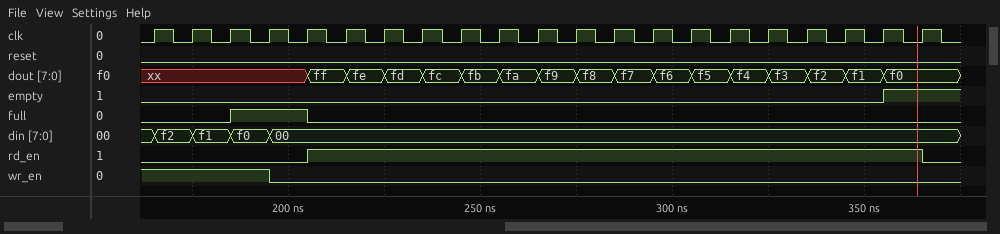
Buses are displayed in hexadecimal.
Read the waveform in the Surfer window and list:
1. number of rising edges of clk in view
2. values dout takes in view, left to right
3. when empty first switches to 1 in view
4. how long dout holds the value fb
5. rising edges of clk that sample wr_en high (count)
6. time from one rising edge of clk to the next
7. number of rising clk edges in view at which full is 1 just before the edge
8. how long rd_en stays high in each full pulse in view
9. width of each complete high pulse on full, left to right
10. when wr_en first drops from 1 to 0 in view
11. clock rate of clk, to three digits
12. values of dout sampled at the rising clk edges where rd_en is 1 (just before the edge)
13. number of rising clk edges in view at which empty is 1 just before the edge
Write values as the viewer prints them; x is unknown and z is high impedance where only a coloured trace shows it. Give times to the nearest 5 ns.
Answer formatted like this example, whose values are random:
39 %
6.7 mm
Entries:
21
xx, ff, fe, fd, fc, fb, fa, f9, f8, f7, f6, f5, f4, f3, f2, f1, f0
355 ns
10 ns
4
10 ns
2
160 ns
20 ns
195 ns
100 MHz
ff, fe, fd, fc, fb, fa, f9, f8, f7, f6, f5, f4, f3, f2, f1, f0
1
